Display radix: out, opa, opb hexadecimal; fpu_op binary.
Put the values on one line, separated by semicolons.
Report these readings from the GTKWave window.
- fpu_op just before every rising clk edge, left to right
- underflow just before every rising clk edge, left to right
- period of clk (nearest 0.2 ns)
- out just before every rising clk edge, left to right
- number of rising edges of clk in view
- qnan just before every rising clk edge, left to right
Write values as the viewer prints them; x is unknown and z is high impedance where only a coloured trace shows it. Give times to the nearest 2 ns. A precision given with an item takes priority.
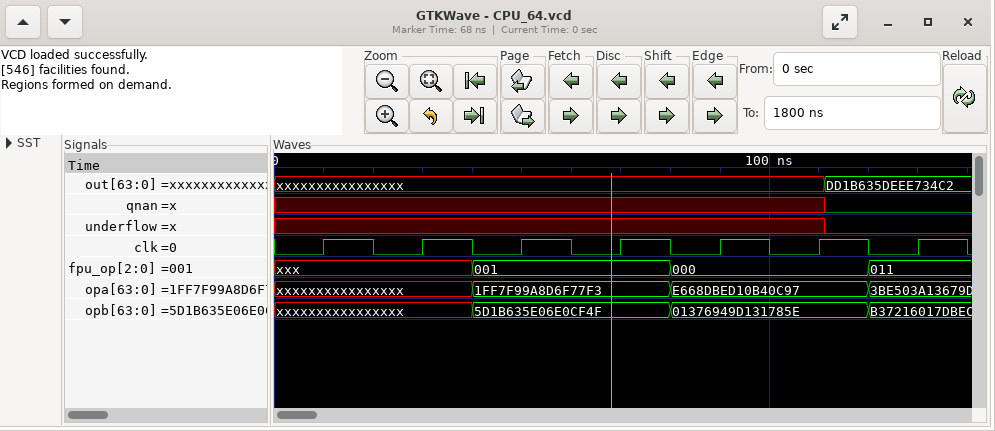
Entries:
xxx, xxx, 001, 001, 000, 000, 011; x x x x x x 0; 20 ns; xxxxxxxxxxxxxxxx, xxxxxxxxxxxxxxxx, xxxxxxxxxxxxxxxx, xxxxxxxxxxxxxxxx, xxxxxxxxxxxxxxxx, xxxxxxxxxxxxxxxx, DD1B635DEEE734C2; 7; x x x x x x 0
